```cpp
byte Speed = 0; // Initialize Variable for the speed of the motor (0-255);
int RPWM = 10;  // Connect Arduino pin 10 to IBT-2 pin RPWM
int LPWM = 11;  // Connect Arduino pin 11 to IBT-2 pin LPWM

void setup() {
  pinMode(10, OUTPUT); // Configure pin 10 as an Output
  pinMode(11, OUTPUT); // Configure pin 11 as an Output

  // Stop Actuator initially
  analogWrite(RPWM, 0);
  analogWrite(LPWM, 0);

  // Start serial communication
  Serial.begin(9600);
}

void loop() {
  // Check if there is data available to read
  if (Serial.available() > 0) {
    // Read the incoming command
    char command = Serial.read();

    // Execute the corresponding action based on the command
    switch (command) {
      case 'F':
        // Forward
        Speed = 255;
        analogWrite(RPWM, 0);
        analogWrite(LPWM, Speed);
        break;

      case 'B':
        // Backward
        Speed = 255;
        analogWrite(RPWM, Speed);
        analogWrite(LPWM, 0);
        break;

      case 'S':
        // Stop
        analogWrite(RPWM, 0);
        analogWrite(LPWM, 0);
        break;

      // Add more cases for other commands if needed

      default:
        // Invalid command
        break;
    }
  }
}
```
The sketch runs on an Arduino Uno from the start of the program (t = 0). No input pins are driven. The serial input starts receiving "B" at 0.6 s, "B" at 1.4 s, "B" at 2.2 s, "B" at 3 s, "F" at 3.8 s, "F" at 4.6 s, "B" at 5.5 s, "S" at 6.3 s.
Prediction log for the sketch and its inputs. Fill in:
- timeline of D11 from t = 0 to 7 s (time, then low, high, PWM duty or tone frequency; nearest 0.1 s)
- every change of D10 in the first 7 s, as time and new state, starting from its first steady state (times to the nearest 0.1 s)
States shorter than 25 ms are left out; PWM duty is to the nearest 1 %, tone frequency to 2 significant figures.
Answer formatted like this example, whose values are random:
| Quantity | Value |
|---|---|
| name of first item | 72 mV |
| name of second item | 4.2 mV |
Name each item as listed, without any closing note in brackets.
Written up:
| Quantity | Value |
|---|---|
| timeline of D11 from t = 0 to 7 s | 0 s low; 3.8 s high; 5.5 s low |
| every change of D10 in the first 7 s, as time and new state, starting from its first steady state | 0 s low; 0.6 s high; 3.8 s low; 5.5 s high; 6.3 s low |
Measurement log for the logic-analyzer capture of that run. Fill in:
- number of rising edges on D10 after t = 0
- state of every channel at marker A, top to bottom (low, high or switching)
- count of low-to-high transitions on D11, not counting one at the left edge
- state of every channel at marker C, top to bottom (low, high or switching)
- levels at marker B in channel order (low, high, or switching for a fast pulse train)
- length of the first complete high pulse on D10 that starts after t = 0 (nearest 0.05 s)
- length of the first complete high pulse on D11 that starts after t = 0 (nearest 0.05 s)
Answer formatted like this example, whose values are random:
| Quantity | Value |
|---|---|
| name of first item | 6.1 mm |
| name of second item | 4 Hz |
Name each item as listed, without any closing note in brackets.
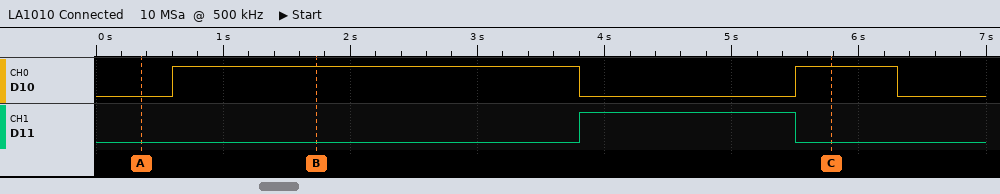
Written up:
| Quantity | Value |
|---|---|
| number of rising edges on D10 after t = 0 | 2 |
| state of every channel at marker A, top to bottom | D10 low, D11 low |
| count of low-to-high transitions on D11, not counting one at the left edge | 1 |
| state of every channel at marker C, top to bottom | D10 high, D11 low |
| levels at marker B in channel order | D10 high, D11 low |
| length of the first complete high pulse on D10 that starts after t = 0 | 3.20 s |
| length of the first complete high pulse on D11 that starts after t = 0 | 1.70 s |
